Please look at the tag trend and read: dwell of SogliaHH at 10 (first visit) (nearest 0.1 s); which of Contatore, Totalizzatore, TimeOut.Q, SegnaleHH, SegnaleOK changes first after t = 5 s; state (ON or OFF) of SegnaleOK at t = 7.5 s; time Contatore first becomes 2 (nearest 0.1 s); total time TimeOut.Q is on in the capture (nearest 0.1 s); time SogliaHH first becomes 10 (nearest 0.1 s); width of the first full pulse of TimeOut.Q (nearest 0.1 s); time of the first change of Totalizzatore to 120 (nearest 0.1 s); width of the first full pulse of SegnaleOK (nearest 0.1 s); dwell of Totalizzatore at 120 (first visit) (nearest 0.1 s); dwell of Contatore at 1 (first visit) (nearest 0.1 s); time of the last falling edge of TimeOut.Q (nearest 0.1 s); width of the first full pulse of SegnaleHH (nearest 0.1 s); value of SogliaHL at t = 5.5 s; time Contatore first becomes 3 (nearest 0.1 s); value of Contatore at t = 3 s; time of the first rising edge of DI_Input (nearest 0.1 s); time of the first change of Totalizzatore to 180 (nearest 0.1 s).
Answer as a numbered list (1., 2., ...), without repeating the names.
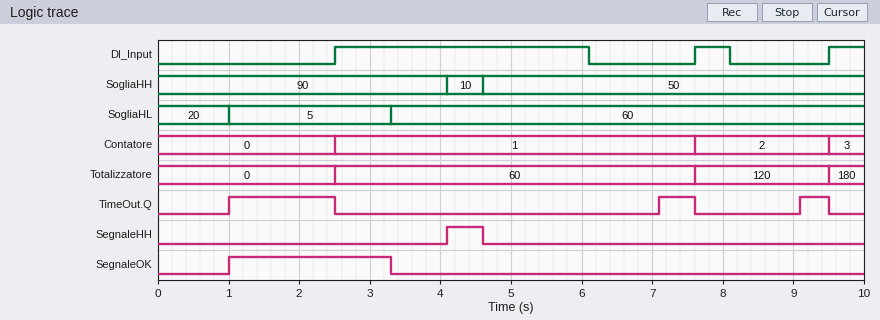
1. 0.5 s
2. TimeOut.Q
3. OFF
4. 7.6 s
5. 2.4 s
6. 4.1 s
7. 1.5 s
8. 7.6 s
9. 2.3 s
10. 1.9 s
11. 5.1 s
12. 9.5 s
13. 0.5 s
14. 60
15. 9.5 s
16. 1
17. 2.5 s
18. 9.5 s
